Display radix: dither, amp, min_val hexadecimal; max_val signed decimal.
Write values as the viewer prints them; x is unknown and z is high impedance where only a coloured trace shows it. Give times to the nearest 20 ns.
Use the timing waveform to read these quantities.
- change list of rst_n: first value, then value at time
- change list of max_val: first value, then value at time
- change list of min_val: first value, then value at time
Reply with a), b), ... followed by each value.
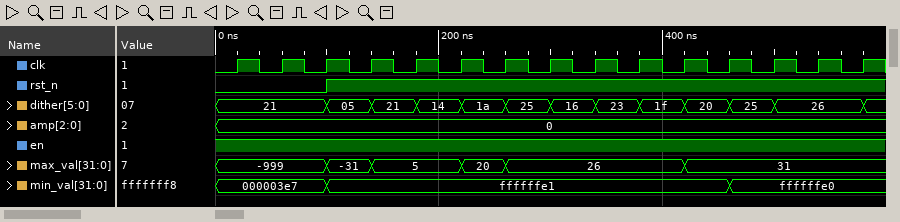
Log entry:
a) 0, 1 at 100 ns
b) -999, -31 at 100 ns, 5 at 140 ns, 20 at 220 ns, 26 at 260 ns, 31 at 420 ns
c) 000003e7, ffffffe1 at 100 ns, ffffffe0 at 460 ns
